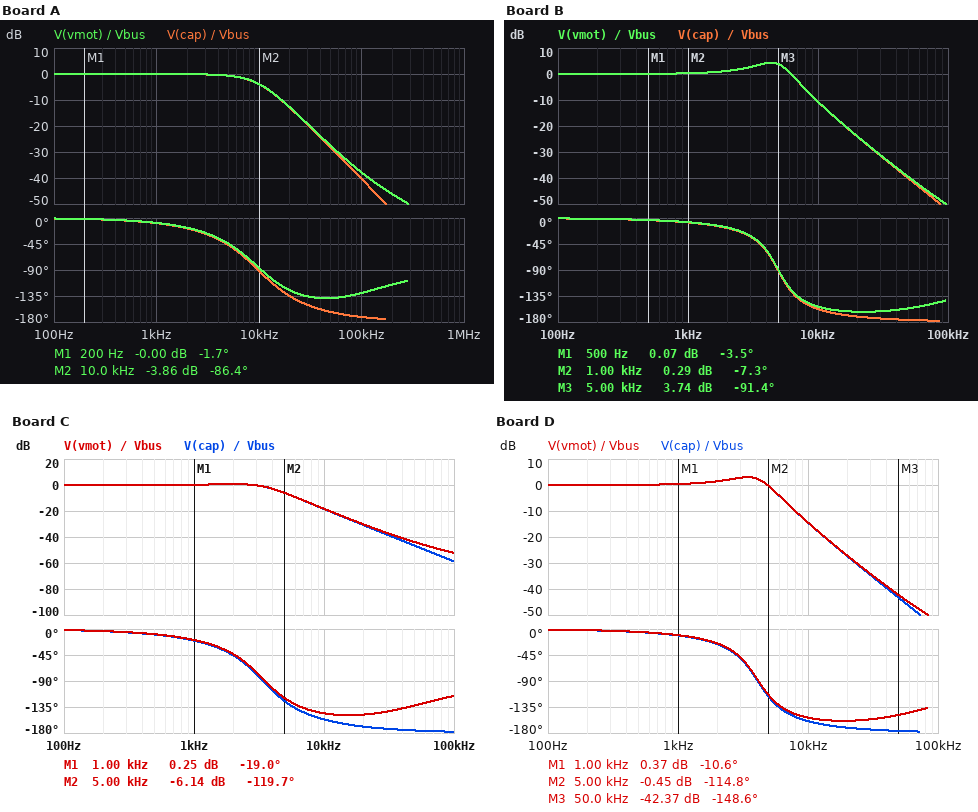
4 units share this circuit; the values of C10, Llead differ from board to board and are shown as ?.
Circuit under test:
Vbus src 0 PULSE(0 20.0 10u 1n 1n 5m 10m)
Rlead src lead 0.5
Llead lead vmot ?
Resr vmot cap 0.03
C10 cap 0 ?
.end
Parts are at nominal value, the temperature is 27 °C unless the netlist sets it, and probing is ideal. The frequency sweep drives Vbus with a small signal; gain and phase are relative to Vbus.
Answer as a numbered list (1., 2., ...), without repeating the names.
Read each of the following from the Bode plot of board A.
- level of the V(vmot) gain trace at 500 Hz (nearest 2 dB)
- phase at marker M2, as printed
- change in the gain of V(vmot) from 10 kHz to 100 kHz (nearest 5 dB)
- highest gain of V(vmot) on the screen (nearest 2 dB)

1. 0 dB
2. -86.4 deg
3. -35 dB
4. 0 dB
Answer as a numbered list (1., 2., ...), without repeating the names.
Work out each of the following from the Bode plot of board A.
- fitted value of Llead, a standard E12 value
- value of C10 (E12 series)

1. 5.6 µH
2. 47 µF
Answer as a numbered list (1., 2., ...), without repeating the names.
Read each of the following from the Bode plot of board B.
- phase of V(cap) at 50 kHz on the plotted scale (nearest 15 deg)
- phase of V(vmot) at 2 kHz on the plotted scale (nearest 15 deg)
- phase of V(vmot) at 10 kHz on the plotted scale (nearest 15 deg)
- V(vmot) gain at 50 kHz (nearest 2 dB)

1. -180 deg
2. -15 deg
3. -150 deg
4. -40 dB
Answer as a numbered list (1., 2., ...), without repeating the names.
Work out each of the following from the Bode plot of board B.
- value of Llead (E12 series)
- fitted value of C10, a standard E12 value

1. 27 µH
2. 39 µF
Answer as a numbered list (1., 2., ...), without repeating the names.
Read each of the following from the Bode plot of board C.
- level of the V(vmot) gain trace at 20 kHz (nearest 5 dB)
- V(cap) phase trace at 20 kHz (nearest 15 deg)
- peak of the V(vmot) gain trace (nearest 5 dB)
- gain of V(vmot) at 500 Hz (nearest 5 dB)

1. -30 dB
2. -165 deg
3. 0 dB
4. 0 dB
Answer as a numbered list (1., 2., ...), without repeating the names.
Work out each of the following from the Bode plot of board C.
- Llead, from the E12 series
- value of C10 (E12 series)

1. 22 µH
2. 100 µF
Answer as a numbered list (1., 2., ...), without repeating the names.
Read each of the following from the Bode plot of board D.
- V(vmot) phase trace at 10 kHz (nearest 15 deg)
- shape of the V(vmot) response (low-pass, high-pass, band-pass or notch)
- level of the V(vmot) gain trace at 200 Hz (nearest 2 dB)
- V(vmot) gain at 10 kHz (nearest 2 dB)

1. -150 deg
2. low-pass
3. 0 dB
4. -14 dB
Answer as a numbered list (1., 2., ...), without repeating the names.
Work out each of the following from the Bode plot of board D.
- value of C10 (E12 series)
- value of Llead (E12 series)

1. 56 µF
2. 27 µH
